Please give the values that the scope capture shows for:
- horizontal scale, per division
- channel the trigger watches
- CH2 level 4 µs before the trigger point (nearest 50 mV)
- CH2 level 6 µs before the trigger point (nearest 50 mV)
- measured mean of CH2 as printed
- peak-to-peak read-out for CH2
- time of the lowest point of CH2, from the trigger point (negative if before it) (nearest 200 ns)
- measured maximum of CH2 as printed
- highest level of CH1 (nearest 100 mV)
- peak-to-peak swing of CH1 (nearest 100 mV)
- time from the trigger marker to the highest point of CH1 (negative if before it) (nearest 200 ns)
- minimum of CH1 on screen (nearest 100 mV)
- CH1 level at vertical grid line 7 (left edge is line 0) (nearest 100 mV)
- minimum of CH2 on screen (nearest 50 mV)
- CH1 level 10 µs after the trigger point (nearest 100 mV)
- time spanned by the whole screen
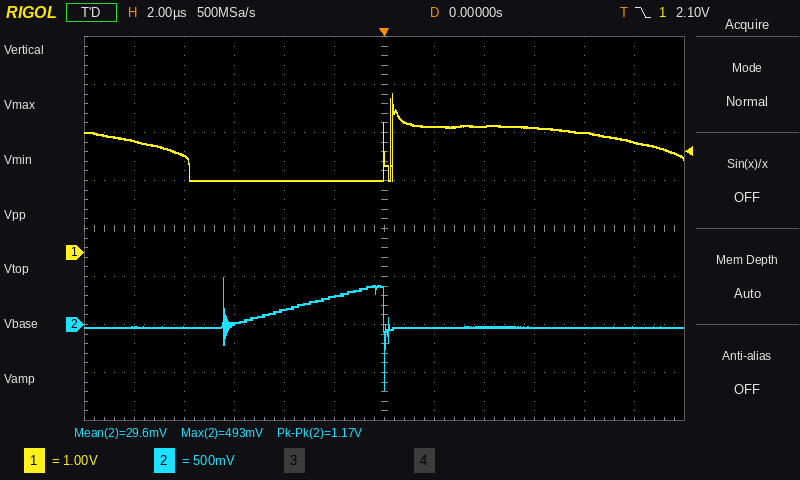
2 µs
CH1
150 mV
0 mV
29.6 mV
1.17 V
0.0 µs
493 mV
3.3 V
1.8 V
+400 ns
1.5 V
2.6 V
-700 mV
2.3 V
24 µs
